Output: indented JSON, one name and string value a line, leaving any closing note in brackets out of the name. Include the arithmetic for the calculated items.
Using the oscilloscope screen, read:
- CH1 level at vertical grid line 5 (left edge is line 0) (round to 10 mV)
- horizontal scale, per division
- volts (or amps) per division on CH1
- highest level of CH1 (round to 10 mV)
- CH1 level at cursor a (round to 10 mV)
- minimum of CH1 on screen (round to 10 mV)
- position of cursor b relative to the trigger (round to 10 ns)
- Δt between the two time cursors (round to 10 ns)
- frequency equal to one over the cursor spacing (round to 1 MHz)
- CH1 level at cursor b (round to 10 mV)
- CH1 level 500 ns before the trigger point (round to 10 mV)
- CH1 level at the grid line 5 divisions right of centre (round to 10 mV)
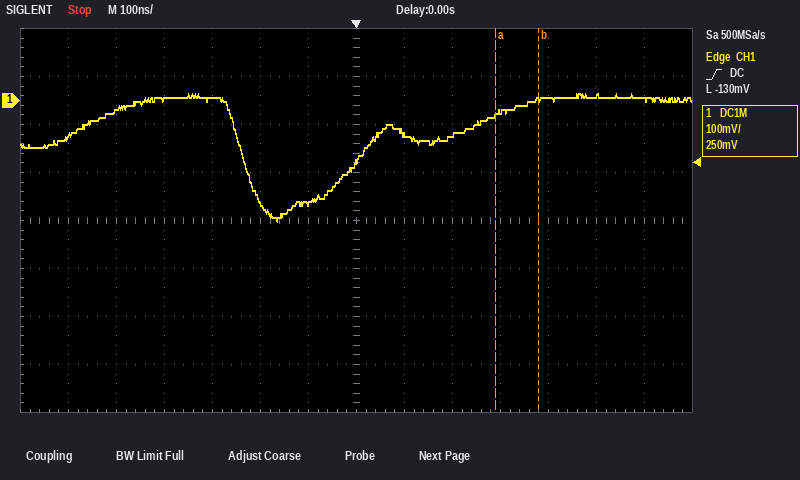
{
  "CH1 level at vertical grid line 5 (left edge is line 0)": "-210 mV",
  "horizontal scale, per division": "100 ns",
  "volts (or amps) per division on CH1": "100 mV",
  "highest level of CH1": "10 mV",
  "CH1 level at cursor a": "-30 mV",
  "minimum of CH1 on screen": "-250 mV",
  "position of cursor b relative to the trigger": "+380 ns",
  "Δt between the two time cursors": "90 ns",
  "frequency equal to one over the cursor spacing": "1 / 90 ns ≈ 11 MHz",
  "CH1 level at cursor b": "0 mV",
  "CH1 level 500 ns before the trigger point": "-20 mV",
  "CH1 level at the grid line 5 divisions right of centre": "10 mV"
}
